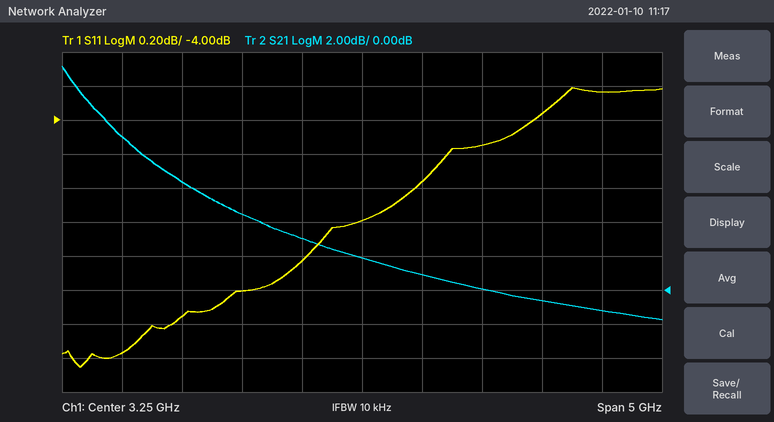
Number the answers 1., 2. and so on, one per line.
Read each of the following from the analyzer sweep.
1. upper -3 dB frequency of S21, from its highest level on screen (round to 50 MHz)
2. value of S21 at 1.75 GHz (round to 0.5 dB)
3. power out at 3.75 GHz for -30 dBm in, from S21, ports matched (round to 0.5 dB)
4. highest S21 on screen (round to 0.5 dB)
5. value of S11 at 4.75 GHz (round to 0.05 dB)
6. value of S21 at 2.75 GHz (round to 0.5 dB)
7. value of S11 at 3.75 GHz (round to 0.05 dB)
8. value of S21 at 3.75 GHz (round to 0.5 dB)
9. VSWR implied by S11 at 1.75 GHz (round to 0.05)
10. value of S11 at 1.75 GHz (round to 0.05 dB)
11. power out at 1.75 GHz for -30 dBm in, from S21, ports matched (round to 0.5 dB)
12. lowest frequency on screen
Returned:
1. 1.10 GHz
2. 6.5 dB
3. -29.0 dBm
4. 13.0 dB
5. -3.95 dB
6. 3.0 dB
7. -4.35 dB
8. 1.0 dB
9. 3.45
10. -5.15 dB
11. -23.5 dBm
12. 750 MHz
